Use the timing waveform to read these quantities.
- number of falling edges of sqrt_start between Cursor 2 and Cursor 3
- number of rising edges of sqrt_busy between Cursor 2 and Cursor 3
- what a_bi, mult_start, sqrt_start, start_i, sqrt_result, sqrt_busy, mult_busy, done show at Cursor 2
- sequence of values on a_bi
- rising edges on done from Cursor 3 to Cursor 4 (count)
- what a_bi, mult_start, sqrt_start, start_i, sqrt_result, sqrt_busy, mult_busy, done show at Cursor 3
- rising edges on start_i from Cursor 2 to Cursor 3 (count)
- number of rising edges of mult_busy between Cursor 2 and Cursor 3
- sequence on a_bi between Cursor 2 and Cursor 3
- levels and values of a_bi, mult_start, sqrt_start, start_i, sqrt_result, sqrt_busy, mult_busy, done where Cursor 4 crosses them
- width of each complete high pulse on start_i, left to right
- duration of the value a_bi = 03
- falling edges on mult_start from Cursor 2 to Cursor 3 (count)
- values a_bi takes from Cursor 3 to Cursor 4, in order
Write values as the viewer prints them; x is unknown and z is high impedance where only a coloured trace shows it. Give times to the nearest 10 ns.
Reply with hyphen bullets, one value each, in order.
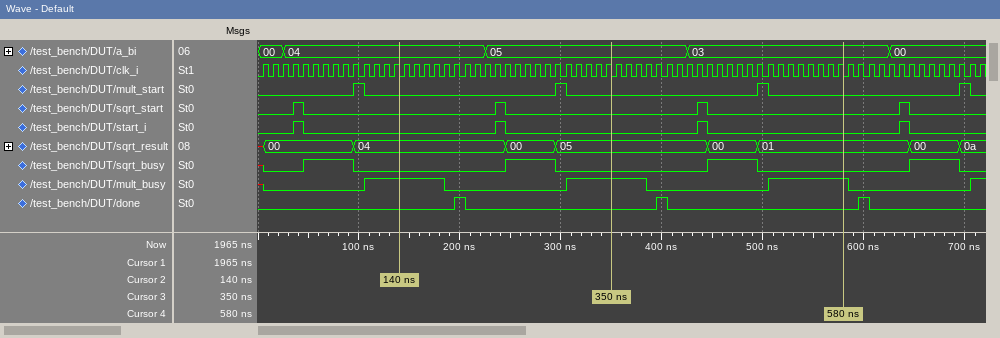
- 1
- 1
- a_bi=04, mult_start=0, sqrt_start=0, start_i=0, sqrt_result=04, sqrt_busy=0, mult_busy=1, done=0
- 00, 04, 05, 03, 00
- 1
- a_bi=05, mult_start=0, sqrt_start=0, start_i=0, sqrt_result=05, sqrt_busy=0, mult_busy=1, done=0
- 1
- 1
- 04, 05
- a_bi=03, mult_start=0, sqrt_start=0, start_i=0, sqrt_result=01, sqrt_busy=0, mult_busy=1, done=0
- 10 ns, 10 ns, 10 ns, 10 ns
- 200 ns
- 1
- 05, 03
